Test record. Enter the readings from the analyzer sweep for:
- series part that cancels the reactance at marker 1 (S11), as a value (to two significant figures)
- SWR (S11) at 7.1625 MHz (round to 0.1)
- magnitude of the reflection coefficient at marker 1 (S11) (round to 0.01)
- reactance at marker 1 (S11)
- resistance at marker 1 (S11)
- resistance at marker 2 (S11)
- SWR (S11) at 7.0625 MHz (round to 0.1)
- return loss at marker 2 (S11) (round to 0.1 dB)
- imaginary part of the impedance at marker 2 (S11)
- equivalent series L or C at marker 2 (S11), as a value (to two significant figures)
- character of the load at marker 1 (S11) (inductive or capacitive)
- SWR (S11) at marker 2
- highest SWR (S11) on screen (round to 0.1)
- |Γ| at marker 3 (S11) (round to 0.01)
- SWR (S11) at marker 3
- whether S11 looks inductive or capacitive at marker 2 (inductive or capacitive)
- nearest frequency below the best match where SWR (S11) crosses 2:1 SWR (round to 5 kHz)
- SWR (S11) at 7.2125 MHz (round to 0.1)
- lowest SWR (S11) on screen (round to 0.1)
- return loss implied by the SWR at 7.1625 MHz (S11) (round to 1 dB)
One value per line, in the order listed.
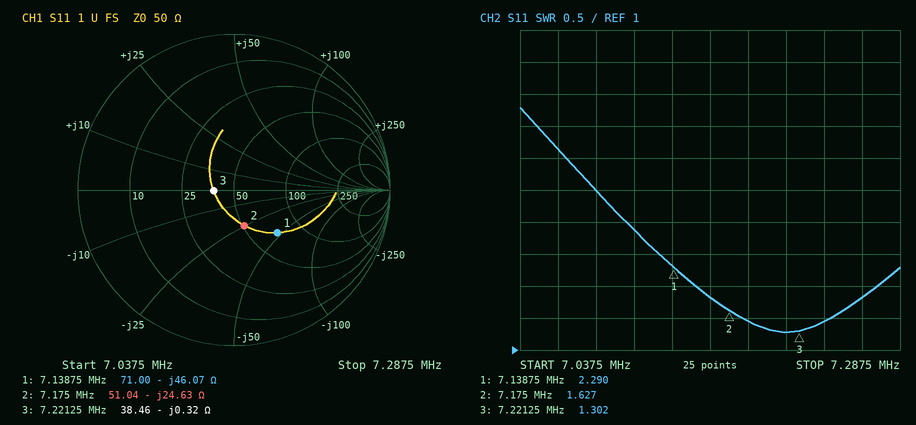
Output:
1.0 µH
1.8
0.39
-46.07 Ω
71.00 Ω
51.04 Ω
4.1
12.5 dB
-24.63 Ω
900 pF
capacitive
1.627
4.8
0.13
1.302
capacitive
7.155 MHz
1.3
1.3
11 dB
